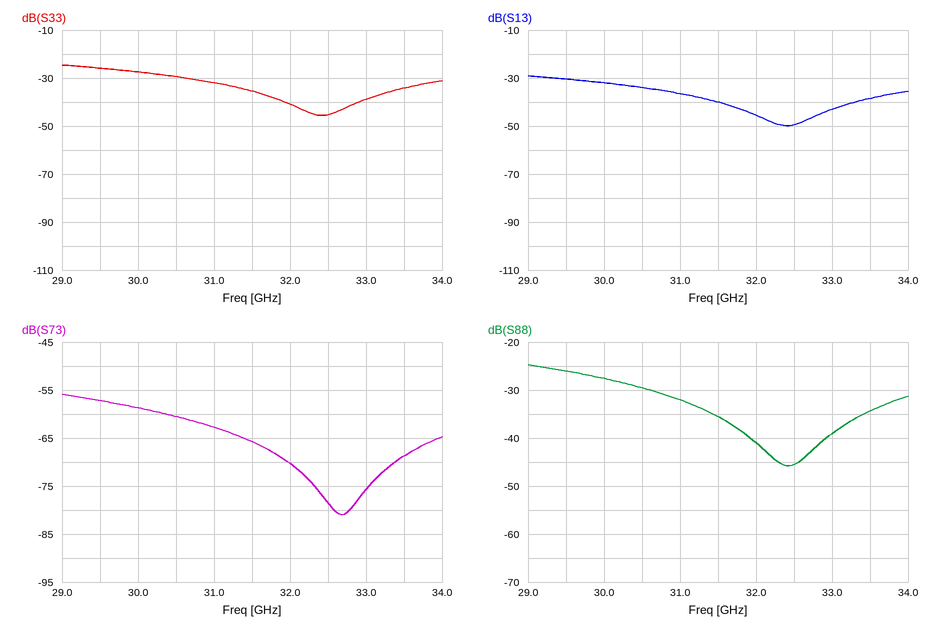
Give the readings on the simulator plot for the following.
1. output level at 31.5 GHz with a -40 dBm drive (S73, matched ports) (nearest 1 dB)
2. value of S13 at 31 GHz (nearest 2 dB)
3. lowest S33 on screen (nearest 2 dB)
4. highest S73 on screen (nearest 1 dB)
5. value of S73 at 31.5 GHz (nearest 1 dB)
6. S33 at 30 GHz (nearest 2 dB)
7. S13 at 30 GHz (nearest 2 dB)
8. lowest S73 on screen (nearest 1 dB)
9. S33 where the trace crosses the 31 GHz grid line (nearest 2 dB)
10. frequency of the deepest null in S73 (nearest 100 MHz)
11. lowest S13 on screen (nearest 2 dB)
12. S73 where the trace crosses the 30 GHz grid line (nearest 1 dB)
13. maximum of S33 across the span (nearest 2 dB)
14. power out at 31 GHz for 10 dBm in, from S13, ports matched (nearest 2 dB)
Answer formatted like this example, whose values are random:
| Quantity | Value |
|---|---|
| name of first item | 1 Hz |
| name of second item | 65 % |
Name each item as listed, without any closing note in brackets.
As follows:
| Quantity | Value |
|---|---|
| output level at 31.5 GHz with a -40 dBm drive (S73, matched ports) | -106 dBm |
| value of S13 at 31 GHz | -36 dB |
| lowest S33 on screen | -46 dB |
| highest S73 on screen | -56 dB |
| value of S73 at 31.5 GHz | -66 dB |
| S33 at 30 GHz | -28 dB |
| S13 at 30 GHz | -32 dB |
| lowest S73 on screen | -81 dB |
| S33 where the trace crosses the 31 GHz grid line | -32 dB |
| frequency of the deepest null in S73 | 32.7 GHz |
| lowest S13 on screen | -50 dB |
| S73 where the trace crosses the 30 GHz grid line | -59 dB |
| maximum of S33 across the span | -24 dB |
| power out at 31 GHz for 10 dBm in, from S13, ports matched | -26 dBm |
